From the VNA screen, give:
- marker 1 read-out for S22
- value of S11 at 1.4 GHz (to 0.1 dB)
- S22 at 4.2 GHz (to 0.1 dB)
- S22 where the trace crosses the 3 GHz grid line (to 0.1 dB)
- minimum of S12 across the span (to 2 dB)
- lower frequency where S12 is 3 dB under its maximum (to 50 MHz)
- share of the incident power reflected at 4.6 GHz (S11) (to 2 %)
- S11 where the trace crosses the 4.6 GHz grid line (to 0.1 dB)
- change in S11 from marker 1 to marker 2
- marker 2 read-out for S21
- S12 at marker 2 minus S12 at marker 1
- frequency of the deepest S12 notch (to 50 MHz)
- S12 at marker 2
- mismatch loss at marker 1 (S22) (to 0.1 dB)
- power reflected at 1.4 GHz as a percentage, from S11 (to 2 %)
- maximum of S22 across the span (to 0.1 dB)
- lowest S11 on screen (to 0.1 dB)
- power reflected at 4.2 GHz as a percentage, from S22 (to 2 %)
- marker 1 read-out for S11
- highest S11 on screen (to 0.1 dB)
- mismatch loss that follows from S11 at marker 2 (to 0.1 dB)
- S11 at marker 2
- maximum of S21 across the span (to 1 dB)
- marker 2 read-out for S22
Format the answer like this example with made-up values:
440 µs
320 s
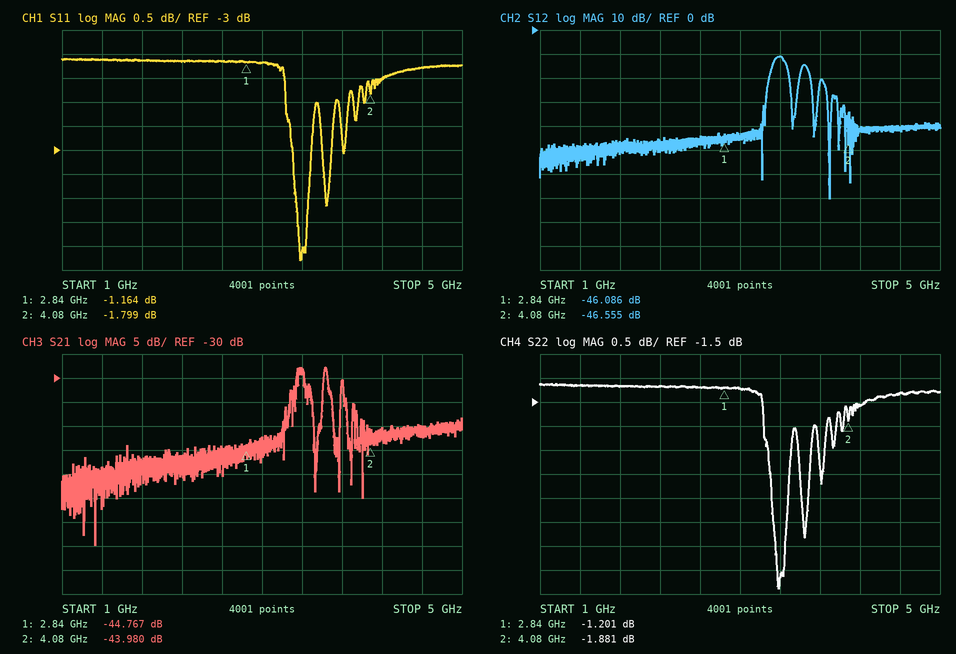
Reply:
-1.201 dB
-1.1 dB
-1.6 dB
-1.2 dB
-70 dB
3.35 GHz
74 %
-1.3 dB
-0.635 dB
-43.980 dB
-0.469 dB
3.90 GHz
-46.555 dB
6.2 dB
78 %
-1.1 dB
-5.3 dB
70 %
-1.164 dB
-1.1 dB
4.7 dB
-1.799 dB
-28 dB
-1.881 dB
